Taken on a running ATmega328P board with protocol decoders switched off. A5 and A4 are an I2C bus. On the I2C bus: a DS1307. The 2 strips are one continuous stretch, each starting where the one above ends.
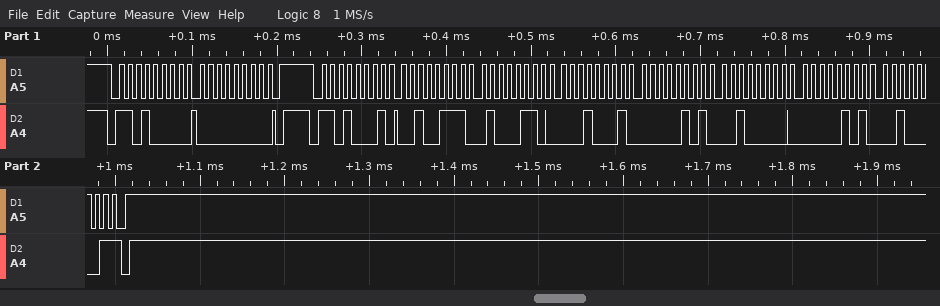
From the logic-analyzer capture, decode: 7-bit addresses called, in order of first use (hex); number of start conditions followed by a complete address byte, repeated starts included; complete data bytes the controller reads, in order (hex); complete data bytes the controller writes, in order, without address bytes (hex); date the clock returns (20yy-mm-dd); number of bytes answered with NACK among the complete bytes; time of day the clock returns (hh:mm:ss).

0x68
2
27 46 11 05 20 05 21
00
2021-05-20
1
11:46:27
